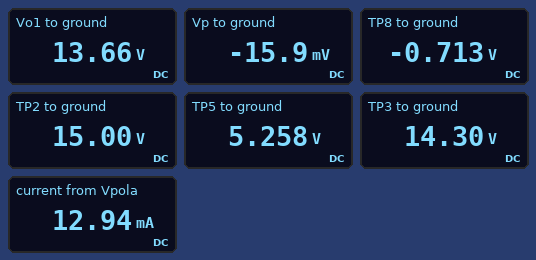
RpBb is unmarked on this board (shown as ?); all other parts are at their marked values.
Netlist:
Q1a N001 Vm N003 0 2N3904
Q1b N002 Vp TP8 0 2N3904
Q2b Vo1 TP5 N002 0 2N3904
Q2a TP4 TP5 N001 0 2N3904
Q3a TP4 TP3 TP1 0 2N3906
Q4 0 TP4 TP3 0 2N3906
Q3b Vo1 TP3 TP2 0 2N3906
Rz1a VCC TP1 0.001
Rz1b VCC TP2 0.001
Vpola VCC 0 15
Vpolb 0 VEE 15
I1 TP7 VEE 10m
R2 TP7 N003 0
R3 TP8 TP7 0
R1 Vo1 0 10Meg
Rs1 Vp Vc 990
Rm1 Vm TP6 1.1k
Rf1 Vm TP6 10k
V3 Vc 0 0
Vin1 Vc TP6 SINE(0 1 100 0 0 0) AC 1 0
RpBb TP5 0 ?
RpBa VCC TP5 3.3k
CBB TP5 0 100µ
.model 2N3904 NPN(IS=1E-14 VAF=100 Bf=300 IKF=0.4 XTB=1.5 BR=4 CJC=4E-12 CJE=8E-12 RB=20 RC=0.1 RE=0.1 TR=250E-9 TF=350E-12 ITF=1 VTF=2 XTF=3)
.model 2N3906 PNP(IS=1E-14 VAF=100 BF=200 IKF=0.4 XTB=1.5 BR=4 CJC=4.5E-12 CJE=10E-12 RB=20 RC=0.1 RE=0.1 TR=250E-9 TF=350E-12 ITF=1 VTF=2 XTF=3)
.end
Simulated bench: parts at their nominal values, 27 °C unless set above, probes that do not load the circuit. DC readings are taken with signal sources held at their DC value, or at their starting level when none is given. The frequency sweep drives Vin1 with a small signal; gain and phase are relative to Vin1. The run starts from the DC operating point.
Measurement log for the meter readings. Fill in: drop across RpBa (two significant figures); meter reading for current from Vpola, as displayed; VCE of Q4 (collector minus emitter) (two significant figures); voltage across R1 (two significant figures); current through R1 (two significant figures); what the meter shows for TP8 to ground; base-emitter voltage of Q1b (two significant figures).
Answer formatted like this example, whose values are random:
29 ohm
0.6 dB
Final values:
9.7 V
12.94 mA
-14 V
14 V
1.4 µA
-0.713 V
700 mV
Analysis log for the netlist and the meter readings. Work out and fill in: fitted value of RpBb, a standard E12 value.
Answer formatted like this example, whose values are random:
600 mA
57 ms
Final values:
1.8 kΩ
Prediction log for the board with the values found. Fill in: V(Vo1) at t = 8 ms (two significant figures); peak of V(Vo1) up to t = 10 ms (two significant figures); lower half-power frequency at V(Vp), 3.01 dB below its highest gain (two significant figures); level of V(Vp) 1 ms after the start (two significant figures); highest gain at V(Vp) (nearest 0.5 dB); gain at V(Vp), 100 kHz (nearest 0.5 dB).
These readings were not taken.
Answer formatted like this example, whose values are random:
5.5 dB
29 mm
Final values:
15 V
15 V
2.3 MHz
-32 mV
-6.5 dB
-14.5 dB
